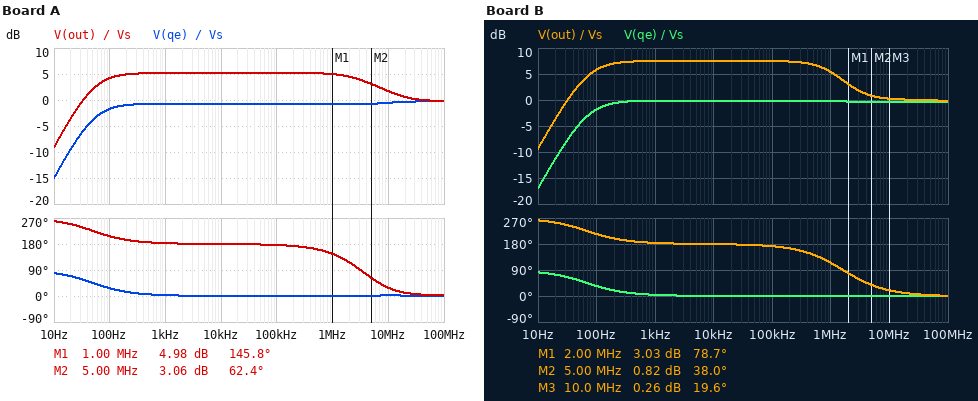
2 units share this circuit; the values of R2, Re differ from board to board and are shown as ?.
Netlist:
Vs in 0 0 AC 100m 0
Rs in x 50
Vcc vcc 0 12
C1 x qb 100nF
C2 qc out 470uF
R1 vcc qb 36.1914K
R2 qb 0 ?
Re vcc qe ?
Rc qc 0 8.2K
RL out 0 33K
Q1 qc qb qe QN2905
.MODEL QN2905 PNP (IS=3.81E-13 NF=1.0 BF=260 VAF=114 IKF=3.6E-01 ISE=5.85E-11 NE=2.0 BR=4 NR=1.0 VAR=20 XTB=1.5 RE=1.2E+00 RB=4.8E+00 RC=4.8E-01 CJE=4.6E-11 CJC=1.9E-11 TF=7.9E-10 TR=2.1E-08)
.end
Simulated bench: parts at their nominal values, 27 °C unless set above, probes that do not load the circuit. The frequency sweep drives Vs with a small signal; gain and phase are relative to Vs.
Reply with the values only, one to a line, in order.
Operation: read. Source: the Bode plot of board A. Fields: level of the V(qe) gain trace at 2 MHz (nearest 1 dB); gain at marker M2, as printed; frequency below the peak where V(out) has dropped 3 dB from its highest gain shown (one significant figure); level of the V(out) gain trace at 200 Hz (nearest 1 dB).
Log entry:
-1 dB
3.06 dB
50 Hz
5 dB
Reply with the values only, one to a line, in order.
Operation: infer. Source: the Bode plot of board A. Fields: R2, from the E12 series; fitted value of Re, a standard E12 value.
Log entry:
470 kΩ
3.3 kΩ
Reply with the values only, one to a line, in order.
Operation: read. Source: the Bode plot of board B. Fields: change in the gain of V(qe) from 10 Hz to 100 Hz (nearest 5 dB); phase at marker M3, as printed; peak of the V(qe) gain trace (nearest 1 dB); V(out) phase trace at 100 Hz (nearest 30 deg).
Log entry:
15 dB
19.6 deg
0 dB
210 deg
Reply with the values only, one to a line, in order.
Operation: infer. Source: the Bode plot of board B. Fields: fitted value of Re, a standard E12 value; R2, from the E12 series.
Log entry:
2.7 kΩ
82 kΩ
